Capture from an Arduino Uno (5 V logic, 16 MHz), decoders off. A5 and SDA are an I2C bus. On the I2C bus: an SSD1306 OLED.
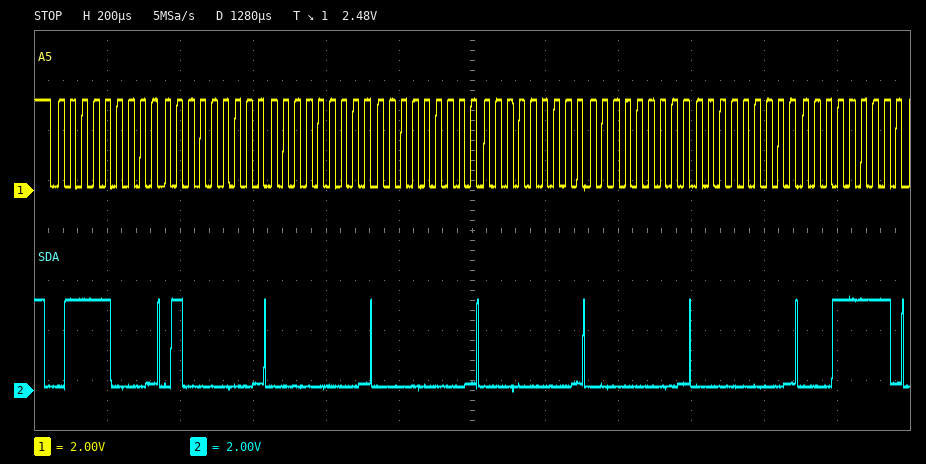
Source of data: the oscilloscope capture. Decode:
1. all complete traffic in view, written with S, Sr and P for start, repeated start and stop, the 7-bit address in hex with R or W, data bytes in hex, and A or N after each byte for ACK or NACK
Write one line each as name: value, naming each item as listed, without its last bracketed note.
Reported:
all complete traffic in view, written with S, Sr and P for start, repeated start and stop, the 7-bit address in hex with R or W, data bytes in hex, and A or N after each byte for ACK or NACK: S 3CW A 40 A 00 A 00 A 00 A 00 A 00 A 1F A
